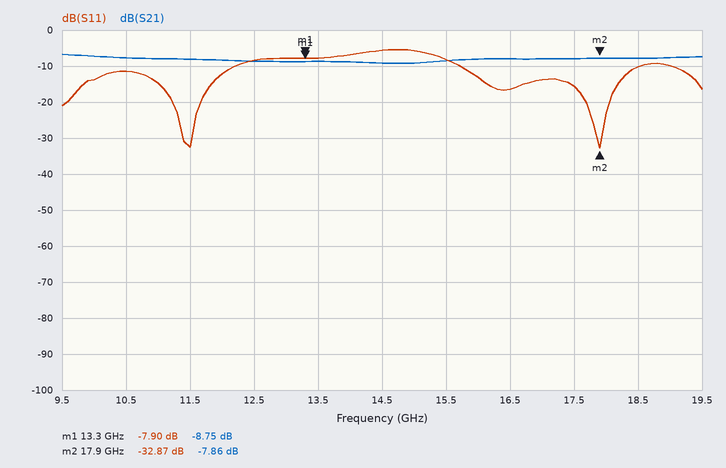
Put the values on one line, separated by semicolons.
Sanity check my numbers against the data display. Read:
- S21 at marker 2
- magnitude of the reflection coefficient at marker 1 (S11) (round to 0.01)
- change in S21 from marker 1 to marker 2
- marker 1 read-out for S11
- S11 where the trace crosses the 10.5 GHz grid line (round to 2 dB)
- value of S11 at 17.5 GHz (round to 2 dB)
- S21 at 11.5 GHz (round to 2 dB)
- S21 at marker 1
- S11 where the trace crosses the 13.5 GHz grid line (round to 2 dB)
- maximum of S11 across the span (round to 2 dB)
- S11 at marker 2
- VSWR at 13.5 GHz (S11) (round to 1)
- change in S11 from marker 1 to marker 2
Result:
-7.86 dB; 0.40; 0.89 dB; -7.90 dB; -12 dB; -16 dB; -8 dB; -8.75 dB; -8 dB; -6 dB; -32.87 dB; 2; -24.97 dB
